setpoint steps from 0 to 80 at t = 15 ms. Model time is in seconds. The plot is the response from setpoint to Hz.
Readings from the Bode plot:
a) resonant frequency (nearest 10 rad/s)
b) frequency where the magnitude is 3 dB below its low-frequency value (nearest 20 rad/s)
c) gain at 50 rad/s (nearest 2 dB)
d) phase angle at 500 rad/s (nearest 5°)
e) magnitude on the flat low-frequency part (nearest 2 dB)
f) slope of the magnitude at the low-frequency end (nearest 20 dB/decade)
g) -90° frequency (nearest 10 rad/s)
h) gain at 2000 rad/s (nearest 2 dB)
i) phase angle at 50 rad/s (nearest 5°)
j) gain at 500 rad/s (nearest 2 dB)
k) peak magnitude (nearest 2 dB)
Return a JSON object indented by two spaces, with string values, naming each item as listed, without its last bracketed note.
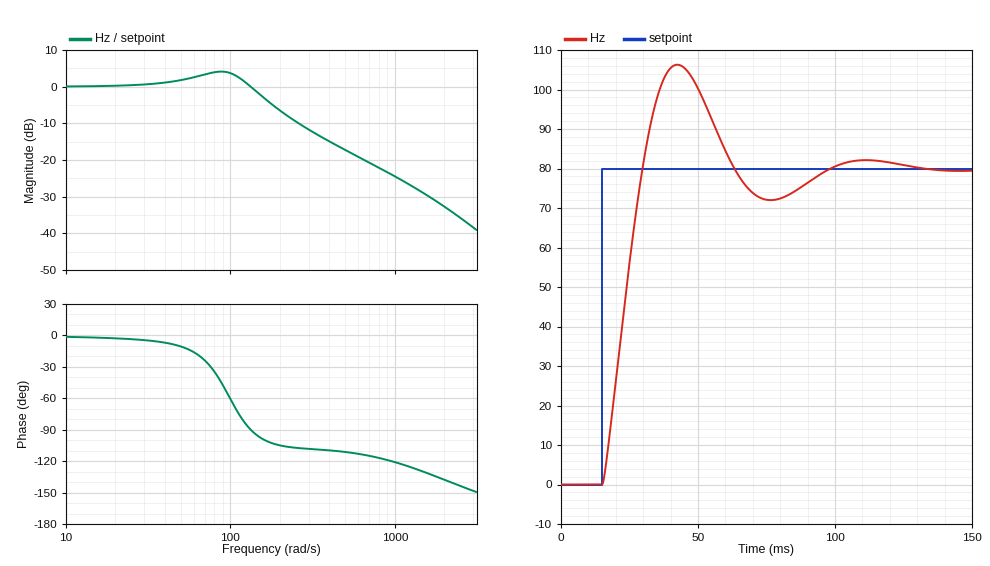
{
  "resonant frequency": "90 rad/s",
  "frequency where the magnitude is 3 dB below its low-frequency value": "160 rad/s",
  "gain at 50 rad/s": "2 dB",
  "phase angle at 500 rad/s": "-110°",
  "magnitude on the flat low-frequency part": "0 dB",
  "slope of the magnitude at the low-frequency end": "0 dB/decade",
  "-90° frequency": "130 rad/s",
  "gain at 2000 rad/s": "-32 dB",
  "phase angle at 50 rad/s": "-10°",
  "gain at 500 rad/s": "-18 dB",
  "peak magnitude": "4 dB"
}
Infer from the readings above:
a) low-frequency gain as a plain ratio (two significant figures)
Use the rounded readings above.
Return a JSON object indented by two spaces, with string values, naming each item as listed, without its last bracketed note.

{
  "low-frequency gain as a plain ratio": "1.0"
}
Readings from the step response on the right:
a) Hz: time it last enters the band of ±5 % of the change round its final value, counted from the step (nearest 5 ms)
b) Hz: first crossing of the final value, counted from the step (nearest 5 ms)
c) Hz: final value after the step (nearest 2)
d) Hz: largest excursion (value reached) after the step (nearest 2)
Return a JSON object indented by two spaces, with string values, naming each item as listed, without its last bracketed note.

{
  "Hz: time it last enters the band of ±5 % of the change round its final value, counted from the step": "75 ms",
  "Hz: first crossing of the final value, counted from the step": "15 ms",
  "Hz: final value after the step": "80",
  "Hz: largest excursion (value reached) after the step": "106"
}
